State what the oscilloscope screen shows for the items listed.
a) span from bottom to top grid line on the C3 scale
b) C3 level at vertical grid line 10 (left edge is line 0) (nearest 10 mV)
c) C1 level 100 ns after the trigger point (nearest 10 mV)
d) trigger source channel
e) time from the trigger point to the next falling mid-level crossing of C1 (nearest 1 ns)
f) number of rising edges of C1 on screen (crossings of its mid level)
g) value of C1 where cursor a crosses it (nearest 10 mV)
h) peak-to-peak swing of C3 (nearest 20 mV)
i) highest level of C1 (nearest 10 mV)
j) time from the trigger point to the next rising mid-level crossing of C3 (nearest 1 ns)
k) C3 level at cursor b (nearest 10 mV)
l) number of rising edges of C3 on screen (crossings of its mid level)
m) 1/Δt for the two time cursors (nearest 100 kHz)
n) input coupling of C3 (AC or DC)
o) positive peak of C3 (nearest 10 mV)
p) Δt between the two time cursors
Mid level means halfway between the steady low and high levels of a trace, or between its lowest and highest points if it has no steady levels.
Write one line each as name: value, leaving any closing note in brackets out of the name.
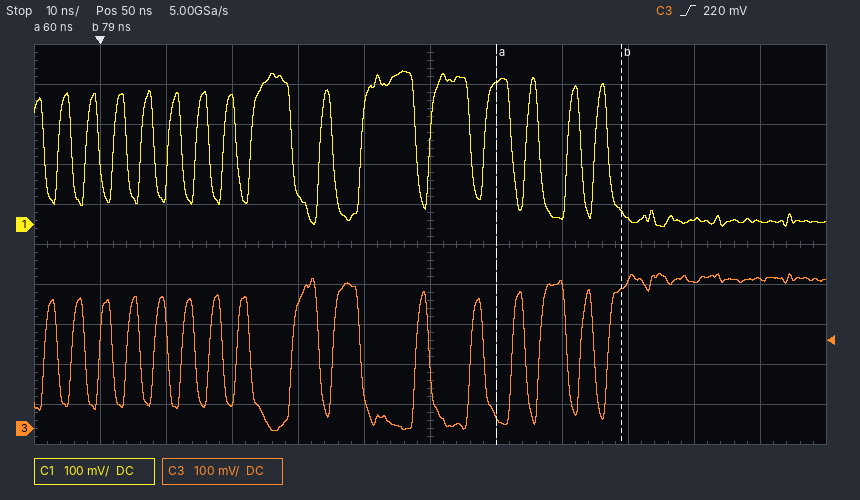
span from bottom to top grid line on the C3 scale: 1 V
C3 level at vertical grid line 10 (left edge is line 0): 370 mV
C1 level 100 ns after the trigger point: 10 mV
trigger source channel: C3
time from the trigger point to the next falling mid-level crossing of C1: 4 ns
number of rising edges of C1 on screen: 15
value of C1 where cursor a crosses it: 360 mV
peak-to-peak swing of C3: 400 mV
highest level of C1: 380 mV
time from the trigger point to the next rising mid-level crossing of C3: 4 ns
C3 level at cursor b: 350 mV
number of rising edges of C3 on screen: 16
1/Δt for the two time cursors: 52.6 MHz
input coupling of C3: DC
positive peak of C3: 390 mV
Δt between the two time cursors: 19 ns
